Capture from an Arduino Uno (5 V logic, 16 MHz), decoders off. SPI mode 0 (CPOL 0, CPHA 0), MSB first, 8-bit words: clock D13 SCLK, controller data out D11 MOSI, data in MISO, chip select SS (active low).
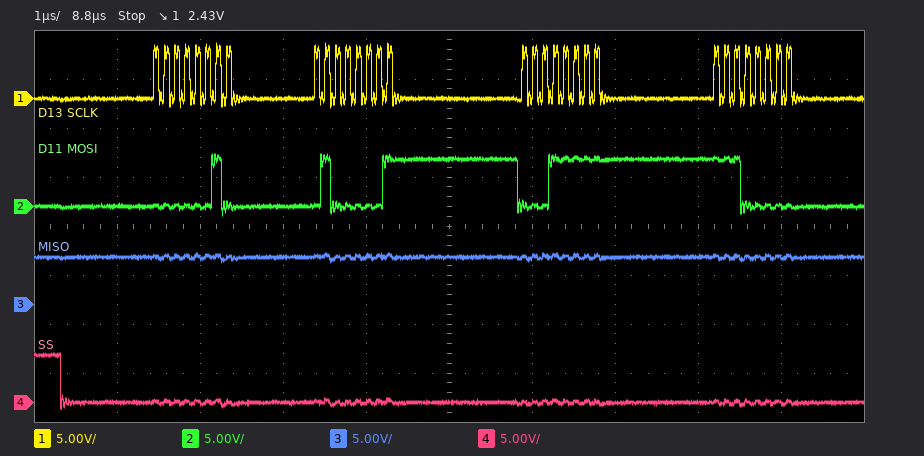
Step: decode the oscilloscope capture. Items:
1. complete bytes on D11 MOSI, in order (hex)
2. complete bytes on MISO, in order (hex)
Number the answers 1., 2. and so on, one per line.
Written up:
1. 02 41 1F E0
2. FF FF FF FF
